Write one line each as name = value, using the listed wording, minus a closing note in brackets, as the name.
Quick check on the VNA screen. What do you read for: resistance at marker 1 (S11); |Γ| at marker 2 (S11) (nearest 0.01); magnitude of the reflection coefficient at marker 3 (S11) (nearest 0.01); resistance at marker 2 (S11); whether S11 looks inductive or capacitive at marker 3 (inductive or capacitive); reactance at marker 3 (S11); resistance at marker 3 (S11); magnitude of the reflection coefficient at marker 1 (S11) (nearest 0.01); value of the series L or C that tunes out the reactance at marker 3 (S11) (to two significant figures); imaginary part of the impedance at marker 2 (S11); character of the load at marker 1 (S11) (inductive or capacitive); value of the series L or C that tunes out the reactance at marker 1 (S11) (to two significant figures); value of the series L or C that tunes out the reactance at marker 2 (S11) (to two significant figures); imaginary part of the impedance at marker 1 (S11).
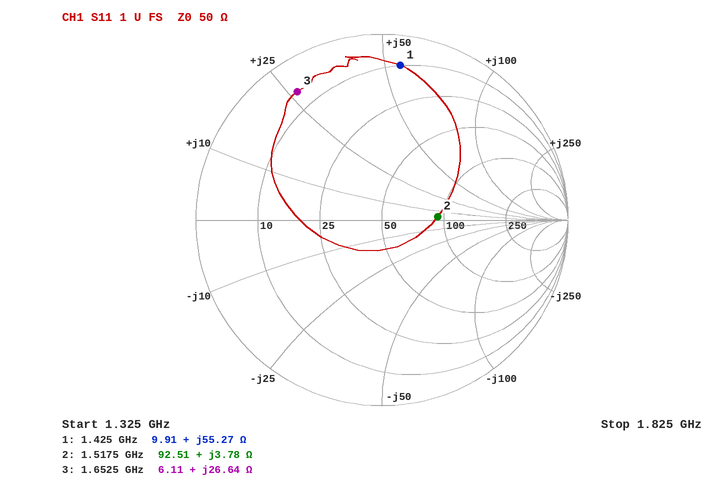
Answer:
resistance at marker 1 = 9.91 Ω
|Γ| at marker 2 (S11) = 0.30
magnitude of the reflection coefficient at marker 3 (S11) = 0.83
resistance at marker 2 = 92.51 Ω
whether S11 looks inductive or capacitive at marker 3 = inductive
reactance at marker 3 = +26.64 Ω
resistance at marker 3 = 6.11 Ω
magnitude of the reflection coefficient at marker 1 (S11) = 0.84
value of the series L or C that tunes out the reactance at marker 3 (S11) = 3.6 pF
imaginary part of the impedance at marker 2 = +3.78 Ω
character of the load at marker 1 (S11) = inductive
value of the series L or C that tunes out the reactance at marker 1 (S11) = 2.0 pF
value of the series L or C that tunes out the reactance at marker 2 (S11) = 28 pF
imaginary part of the impedance at marker 1 = +55.27 Ω
